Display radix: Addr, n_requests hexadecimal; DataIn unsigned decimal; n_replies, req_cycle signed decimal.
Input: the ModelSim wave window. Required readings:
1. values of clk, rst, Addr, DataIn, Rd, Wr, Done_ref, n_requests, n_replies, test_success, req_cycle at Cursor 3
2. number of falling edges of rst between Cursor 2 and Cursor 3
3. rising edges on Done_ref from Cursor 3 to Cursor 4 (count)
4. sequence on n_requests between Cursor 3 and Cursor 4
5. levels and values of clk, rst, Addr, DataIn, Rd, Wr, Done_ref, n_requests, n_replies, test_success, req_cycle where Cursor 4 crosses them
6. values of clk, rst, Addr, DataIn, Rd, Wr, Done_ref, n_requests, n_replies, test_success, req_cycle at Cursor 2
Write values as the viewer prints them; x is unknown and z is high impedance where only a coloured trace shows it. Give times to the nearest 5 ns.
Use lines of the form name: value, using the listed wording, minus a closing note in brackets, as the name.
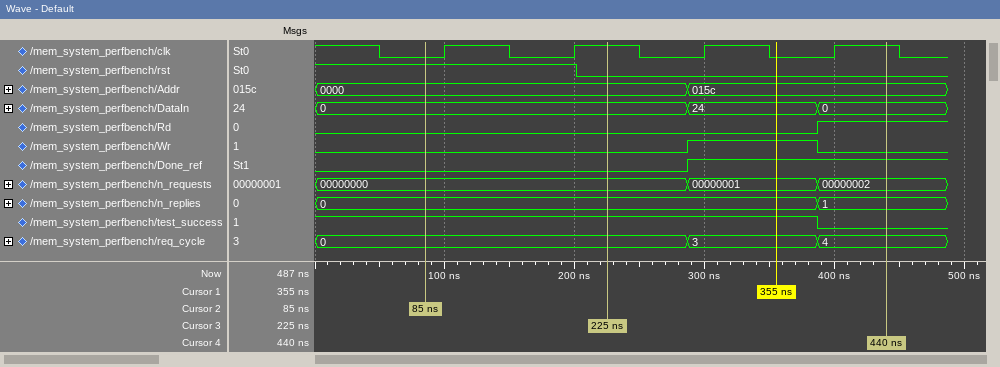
values of clk, rst, Addr, DataIn, Rd, Wr, Done_ref, n_requests, n_replies, test_success, req_cycle at Cursor 3: clk=1, rst=0, Addr=0000, DataIn=0, Rd=0, Wr=0, Done_ref=0, n_requests=00000000, n_replies=0, test_success=1, req_cycle=0
number of falling edges of rst between Cursor 2 and Cursor 3: 1
rising edges on Done_ref from Cursor 3 to Cursor 4: 1
sequence on n_requests between Cursor 3 and Cursor 4: 00000000, 00000001, 00000002
levels and values of clk, rst, Addr, DataIn, Rd, Wr, Done_ref, n_requests, n_replies, test_success, req_cycle where Cursor 4 crosses them: clk=1, rst=0, Addr=015c, DataIn=0, Rd=1, Wr=0, Done_ref=1, n_requests=00000002, n_replies=1, test_success=0, req_cycle=4
values of clk, rst, Addr, DataIn, Rd, Wr, Done_ref, n_requests, n_replies, test_success, req_cycle at Cursor 2: clk=0, rst=1, Addr=0000, DataIn=0, Rd=0, Wr=0, Done_ref=0, n_requests=00000000, n_replies=0, test_success=1, req_cycle=0
